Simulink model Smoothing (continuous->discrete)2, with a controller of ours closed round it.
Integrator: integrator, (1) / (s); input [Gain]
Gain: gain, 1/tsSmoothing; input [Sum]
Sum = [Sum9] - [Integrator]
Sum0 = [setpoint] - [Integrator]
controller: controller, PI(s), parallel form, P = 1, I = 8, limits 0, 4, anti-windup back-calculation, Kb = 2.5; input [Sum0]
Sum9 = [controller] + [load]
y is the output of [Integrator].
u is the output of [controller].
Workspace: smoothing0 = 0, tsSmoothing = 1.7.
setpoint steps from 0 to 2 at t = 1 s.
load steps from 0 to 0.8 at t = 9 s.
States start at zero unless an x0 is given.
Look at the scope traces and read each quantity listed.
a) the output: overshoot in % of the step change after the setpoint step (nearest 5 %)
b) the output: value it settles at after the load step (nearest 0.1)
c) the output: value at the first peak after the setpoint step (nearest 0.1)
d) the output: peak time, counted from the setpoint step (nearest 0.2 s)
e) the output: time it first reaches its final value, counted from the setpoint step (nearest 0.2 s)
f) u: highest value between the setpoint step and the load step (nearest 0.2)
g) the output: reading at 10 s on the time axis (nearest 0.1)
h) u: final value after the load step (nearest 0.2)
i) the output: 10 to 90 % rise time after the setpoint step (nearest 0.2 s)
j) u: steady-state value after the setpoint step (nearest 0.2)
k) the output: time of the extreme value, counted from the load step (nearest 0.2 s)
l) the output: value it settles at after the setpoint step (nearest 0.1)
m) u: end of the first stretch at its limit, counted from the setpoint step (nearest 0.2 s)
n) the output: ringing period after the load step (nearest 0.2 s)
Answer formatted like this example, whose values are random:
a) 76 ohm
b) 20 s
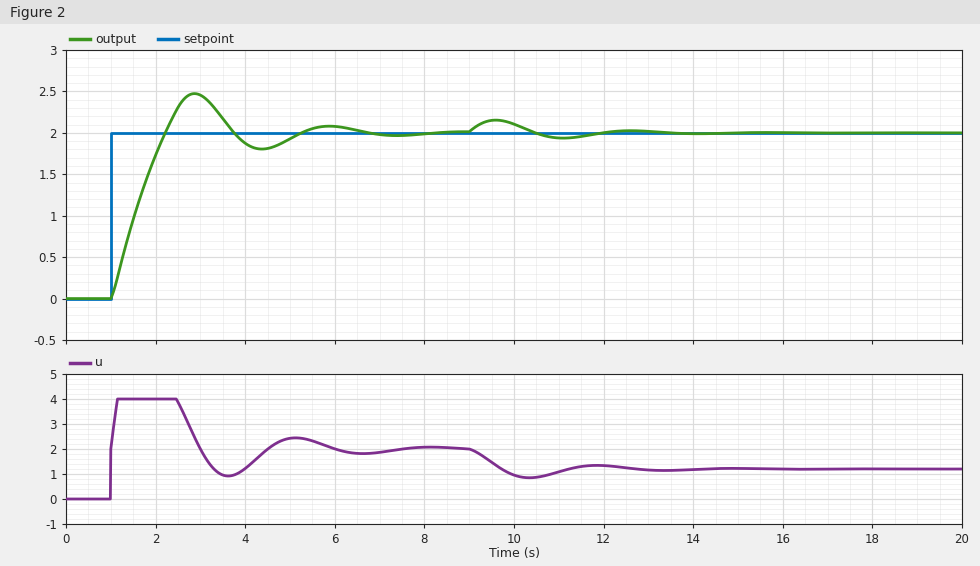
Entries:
a) 25 %
b) 2.0
c) 2.5
d) 1.8 s
e) 1.2 s
f) 4.0
g) 2.1
h) 1.2
i) 1.0 s
j) 2.0
k) 0.6 s
l) 2.0
m) 1.4 s
n) 3.0 s
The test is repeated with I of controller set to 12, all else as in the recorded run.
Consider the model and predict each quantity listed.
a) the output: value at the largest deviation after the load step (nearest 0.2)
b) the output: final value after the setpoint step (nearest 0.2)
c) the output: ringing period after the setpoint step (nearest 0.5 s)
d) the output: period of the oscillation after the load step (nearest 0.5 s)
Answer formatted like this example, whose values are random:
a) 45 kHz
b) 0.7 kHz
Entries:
a) 2.2
b) 2.0
c) 2.5 s
d) 2.5 s
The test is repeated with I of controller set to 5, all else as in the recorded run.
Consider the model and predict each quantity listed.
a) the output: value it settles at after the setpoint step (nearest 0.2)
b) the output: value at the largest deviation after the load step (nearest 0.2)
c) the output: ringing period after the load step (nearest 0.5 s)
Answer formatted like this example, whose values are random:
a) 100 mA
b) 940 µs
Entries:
a) 2.0
b) 2.2
c) 4.0 s
